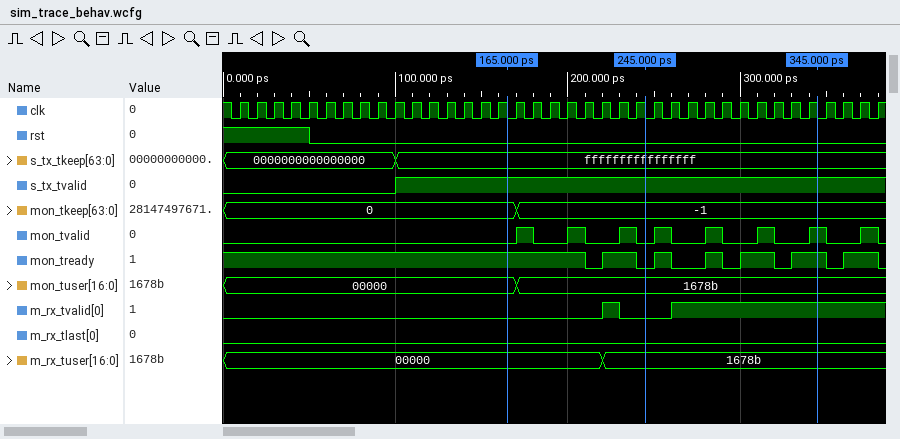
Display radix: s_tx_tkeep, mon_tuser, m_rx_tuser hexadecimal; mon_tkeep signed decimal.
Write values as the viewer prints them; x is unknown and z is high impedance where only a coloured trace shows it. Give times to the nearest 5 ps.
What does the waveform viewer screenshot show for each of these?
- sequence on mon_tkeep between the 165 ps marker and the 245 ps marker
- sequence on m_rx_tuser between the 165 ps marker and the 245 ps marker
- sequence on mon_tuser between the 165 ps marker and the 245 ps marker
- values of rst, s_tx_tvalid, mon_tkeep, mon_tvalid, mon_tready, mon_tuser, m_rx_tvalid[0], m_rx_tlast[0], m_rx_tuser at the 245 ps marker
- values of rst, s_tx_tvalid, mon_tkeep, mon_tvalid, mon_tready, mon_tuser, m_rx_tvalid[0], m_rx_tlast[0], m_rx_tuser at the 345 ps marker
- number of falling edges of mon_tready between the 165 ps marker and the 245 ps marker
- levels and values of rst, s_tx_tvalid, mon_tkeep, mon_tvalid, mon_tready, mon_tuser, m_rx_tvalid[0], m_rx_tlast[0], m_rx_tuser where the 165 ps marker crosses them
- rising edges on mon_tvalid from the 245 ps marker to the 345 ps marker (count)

0, -1
00000, 1678b
00000, 1678b
rst=0, s_tx_tvalid=1, mon_tkeep=-1, mon_tvalid=0, mon_tready=0, mon_tuser=1678b, m_rx_tvalid[0]=0, m_rx_tlast[0]=0, m_rx_tuser=1678b
rst=0, s_tx_tvalid=1, mon_tkeep=-1, mon_tvalid=1, mon_tready=1, mon_tuser=1678b, m_rx_tvalid[0]=1, m_rx_tlast[0]=0, m_rx_tuser=1678b
2
rst=0, s_tx_tvalid=1, mon_tkeep=0, mon_tvalid=0, mon_tready=1, mon_tuser=00000, m_rx_tvalid[0]=0, m_rx_tlast[0]=0, m_rx_tuser=00000
4
